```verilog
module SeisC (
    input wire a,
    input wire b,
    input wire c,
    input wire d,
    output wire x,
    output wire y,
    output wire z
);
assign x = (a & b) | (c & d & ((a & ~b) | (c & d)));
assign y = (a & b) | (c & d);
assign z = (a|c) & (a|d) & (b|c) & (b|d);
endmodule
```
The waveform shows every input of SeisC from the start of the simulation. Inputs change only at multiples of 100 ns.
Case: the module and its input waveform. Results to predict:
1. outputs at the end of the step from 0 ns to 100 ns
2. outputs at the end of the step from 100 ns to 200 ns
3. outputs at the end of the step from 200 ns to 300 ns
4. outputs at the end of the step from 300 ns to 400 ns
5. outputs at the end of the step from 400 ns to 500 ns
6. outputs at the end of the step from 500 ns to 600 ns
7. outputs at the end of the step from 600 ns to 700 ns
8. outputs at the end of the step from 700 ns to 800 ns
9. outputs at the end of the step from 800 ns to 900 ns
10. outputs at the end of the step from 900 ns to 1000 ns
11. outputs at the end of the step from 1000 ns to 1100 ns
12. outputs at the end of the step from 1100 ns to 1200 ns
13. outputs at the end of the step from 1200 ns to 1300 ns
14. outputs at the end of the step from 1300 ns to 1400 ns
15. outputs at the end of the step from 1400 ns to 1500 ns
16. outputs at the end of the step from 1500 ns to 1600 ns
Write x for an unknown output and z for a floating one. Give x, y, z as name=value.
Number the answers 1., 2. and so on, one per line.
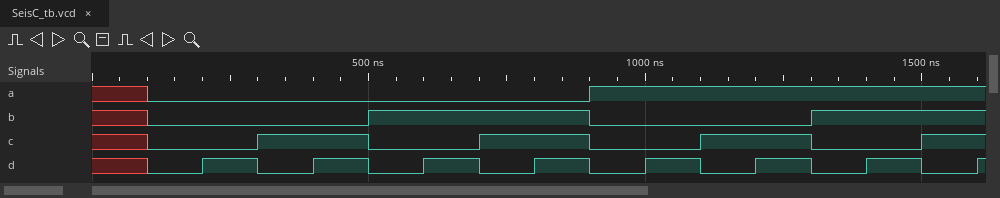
1. x=x, y=x, z=x
2. x=0, y=0, z=0
3. x=0, y=0, z=0
4. x=0, y=0, z=0
5. x=1, y=1, z=1
6. x=0, y=0, z=0
7. x=0, y=0, z=0
8. x=0, y=0, z=0
9. x=1, y=1, z=1
10. x=0, y=0, z=0
11. x=0, y=0, z=0
12. x=0, y=0, z=0
13. x=1, y=1, z=1
14. x=1, y=1, z=1
15. x=1, y=1, z=1
16. x=1, y=1, z=1
